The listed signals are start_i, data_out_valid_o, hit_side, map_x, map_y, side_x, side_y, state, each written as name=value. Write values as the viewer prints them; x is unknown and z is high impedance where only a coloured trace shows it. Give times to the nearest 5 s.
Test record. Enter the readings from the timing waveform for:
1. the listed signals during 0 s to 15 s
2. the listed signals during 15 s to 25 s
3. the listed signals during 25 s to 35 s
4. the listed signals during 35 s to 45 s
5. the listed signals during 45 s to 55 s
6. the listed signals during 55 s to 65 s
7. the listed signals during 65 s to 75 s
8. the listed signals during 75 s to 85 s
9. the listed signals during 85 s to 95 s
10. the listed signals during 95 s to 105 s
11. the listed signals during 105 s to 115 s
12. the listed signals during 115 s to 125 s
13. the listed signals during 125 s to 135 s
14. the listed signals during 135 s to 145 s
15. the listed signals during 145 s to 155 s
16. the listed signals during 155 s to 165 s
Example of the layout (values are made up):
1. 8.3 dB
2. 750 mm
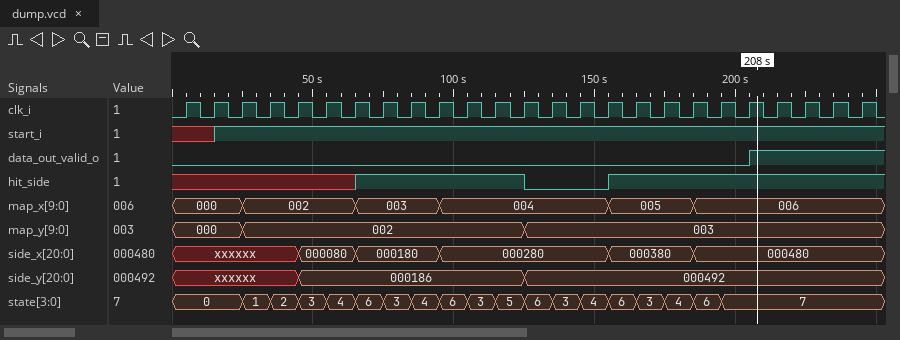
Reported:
1. start_i=x, data_out_valid_o=0, hit_side=x, map_x=000, map_y=000, side_x=xxxxxx, side_y=xxxxxx, state=0
2. start_i=1, data_out_valid_o=0, hit_side=x, map_x=000, map_y=000, side_x=xxxxxx, side_y=xxxxxx, state=0
3. start_i=1, data_out_valid_o=0, hit_side=x, map_x=002, map_y=002, side_x=xxxxxx, side_y=xxxxxx, state=1
4. start_i=1, data_out_valid_o=0, hit_side=x, map_x=002, map_y=002, side_x=xxxxxx, side_y=xxxxxx, state=2
5. start_i=1, data_out_valid_o=0, hit_side=x, map_x=002, map_y=002, side_x=000080, side_y=000186, state=3
6. start_i=1, data_out_valid_o=0, hit_side=x, map_x=002, map_y=002, side_x=000080, side_y=000186, state=4
7. start_i=1, data_out_valid_o=0, hit_side=1, map_x=003, map_y=002, side_x=000180, side_y=000186, state=6
8. start_i=1, data_out_valid_o=0, hit_side=1, map_x=003, map_y=002, side_x=000180, side_y=000186, state=3
9. start_i=1, data_out_valid_o=0, hit_side=1, map_x=003, map_y=002, side_x=000180, side_y=000186, state=4
10. start_i=1, data_out_valid_o=0, hit_side=1, map_x=004, map_y=002, side_x=000280, side_y=000186, state=6
11. start_i=1, data_out_valid_o=0, hit_side=1, map_x=004, map_y=002, side_x=000280, side_y=000186, state=3
12. start_i=1, data_out_valid_o=0, hit_side=1, map_x=004, map_y=002, side_x=000280, side_y=000186, state=5
13. start_i=1, data_out_valid_o=0, hit_side=0, map_x=004, map_y=003, side_x=000280, side_y=000492, state=6
14. start_i=1, data_out_valid_o=0, hit_side=0, map_x=004, map_y=003, side_x=000280, side_y=000492, state=3
15. start_i=1, data_out_valid_o=0, hit_side=0, map_x=004, map_y=003, side_x=000280, side_y=000492, state=4
16. start_i=1, data_out_valid_o=0, hit_side=1, map_x=005, map_y=003, side_x=000380, side_y=000492, state=6
